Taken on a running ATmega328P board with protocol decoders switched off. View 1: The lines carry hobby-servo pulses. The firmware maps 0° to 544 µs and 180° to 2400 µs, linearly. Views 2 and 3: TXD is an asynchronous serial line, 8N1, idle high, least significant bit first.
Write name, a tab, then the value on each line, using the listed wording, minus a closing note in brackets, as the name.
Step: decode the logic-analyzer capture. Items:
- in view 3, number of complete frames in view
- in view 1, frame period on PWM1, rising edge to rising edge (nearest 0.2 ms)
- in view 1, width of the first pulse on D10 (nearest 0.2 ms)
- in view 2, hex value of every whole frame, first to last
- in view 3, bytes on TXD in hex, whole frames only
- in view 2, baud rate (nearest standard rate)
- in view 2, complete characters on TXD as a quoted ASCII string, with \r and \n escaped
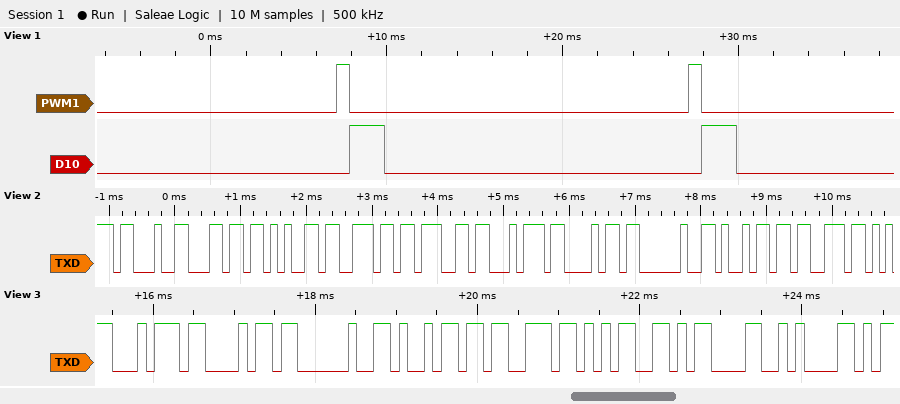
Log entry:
in view 3, number of complete frames in view	8
in view 1, frame period on PWM1, rising edge to rising edge	20.0 ms
in view 1, width of the first pulse on D10	2.0 ms
in view 2, hex value of every whole frame, first to last	23 6C 65 6E 67 74 68 20 69 73
in view 3, bytes on TXD in hex, whole frames only	74 68 20 69 73 35 0D 0A
in view 2, baud rate	9600 baud
in view 2, complete characters on TXD as a quoted ASCII string, with \r and \n escaped	"#length is"
